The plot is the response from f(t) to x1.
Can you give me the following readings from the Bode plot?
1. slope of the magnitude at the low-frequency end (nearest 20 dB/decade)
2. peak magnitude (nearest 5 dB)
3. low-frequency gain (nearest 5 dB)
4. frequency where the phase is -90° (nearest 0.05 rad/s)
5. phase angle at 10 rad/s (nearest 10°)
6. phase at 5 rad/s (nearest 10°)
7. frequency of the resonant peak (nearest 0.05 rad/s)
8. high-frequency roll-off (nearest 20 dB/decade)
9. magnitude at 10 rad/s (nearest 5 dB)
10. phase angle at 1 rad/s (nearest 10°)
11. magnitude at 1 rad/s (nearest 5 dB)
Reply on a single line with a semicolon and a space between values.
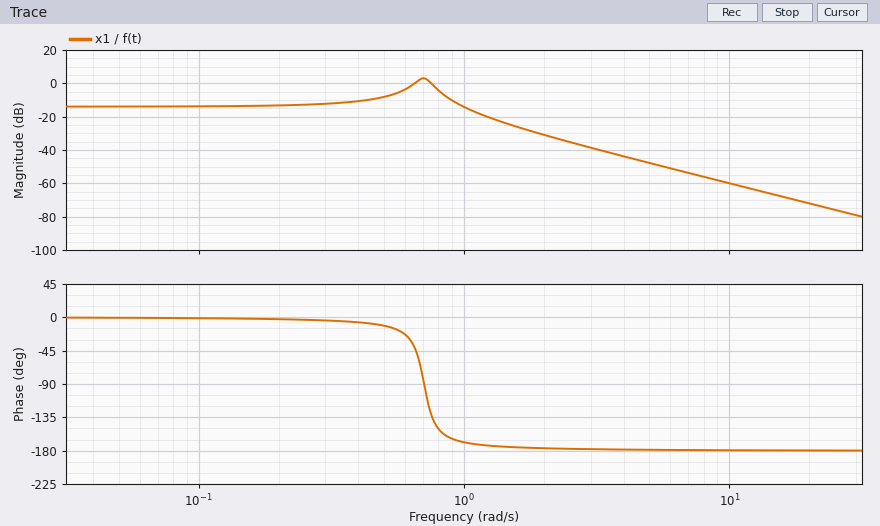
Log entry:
0 dB/decade; 5 dB; -15 dB; 0.70 rad/s; -180°; -180°; 0.70 rad/s; -40 dB/decade; -60 dB; -170°; -15 dB
